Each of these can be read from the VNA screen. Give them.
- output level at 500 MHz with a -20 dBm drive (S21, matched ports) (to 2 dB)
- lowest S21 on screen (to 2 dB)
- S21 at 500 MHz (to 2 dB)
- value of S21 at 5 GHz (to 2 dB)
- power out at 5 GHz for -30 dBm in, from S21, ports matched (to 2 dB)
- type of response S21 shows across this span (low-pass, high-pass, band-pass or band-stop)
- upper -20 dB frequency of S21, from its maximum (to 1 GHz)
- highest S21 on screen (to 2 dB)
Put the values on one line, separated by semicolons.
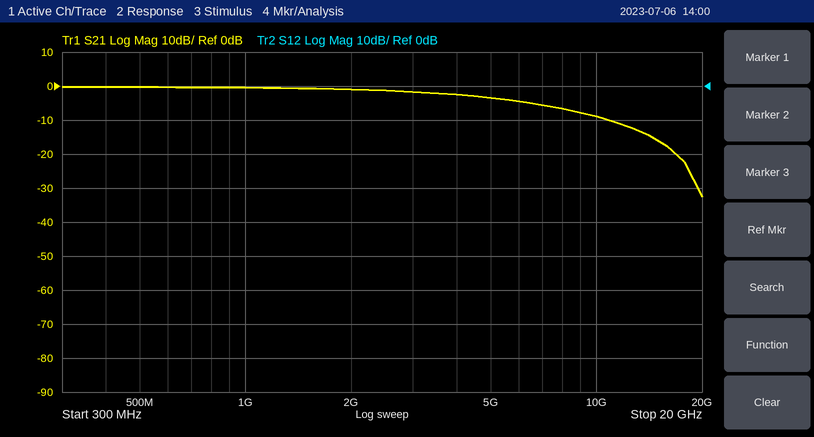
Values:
-20 dBm; -32 dB; 0 dB; -4 dB; -34 dBm; low-pass; 17 GHz; 0 dB
